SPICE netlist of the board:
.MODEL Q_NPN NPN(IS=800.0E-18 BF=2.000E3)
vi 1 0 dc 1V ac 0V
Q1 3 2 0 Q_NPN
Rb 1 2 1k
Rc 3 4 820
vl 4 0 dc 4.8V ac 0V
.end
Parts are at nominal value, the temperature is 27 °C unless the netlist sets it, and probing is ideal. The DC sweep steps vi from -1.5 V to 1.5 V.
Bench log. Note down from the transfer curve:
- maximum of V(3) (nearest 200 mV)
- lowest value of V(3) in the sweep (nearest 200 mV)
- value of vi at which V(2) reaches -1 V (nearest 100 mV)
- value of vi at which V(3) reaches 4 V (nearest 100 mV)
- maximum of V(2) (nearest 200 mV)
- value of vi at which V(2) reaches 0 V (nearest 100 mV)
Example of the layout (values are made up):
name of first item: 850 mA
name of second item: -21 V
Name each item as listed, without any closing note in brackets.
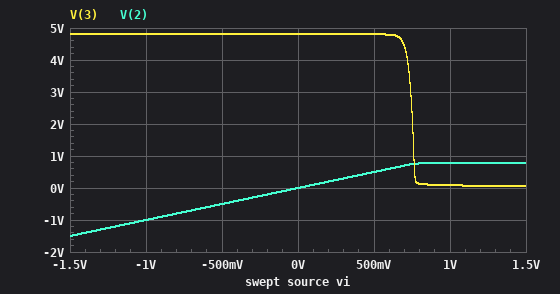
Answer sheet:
maximum of V(3): 4.8 V
lowest value of V(3) in the sweep: 0 V
value of vi at which V(2) reaches -1 V: -1.0 V
value of vi at which V(3) reaches 4 V: 700 mV
maximum of V(2): 800 mV
value of vi at which V(2) reaches 0 V: 0 V
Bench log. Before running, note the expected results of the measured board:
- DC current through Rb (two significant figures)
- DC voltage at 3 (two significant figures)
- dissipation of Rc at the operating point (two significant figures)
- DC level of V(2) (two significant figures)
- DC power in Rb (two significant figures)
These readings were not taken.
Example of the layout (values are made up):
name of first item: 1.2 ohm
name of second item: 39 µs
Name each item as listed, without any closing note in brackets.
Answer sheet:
DC current through Rb: 230 µA
DC voltage at 3: 85 mV
dissipation of Rc at the operating point: 27 mW
DC level of V(2): 770 mV
DC power in Rb: 54 µW
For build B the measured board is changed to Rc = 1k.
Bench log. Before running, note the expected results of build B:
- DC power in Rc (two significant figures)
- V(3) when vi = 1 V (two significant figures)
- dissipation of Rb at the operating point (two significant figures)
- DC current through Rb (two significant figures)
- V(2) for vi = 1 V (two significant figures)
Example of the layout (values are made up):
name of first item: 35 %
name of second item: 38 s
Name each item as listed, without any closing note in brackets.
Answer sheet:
DC power in Rc: 22 mW
V(3) when vi = 1 V: 80 mV
dissipation of Rb at the operating point: 56 µW
DC current through Rb: 240 µA
V(2) for vi = 1 V: 760 mV
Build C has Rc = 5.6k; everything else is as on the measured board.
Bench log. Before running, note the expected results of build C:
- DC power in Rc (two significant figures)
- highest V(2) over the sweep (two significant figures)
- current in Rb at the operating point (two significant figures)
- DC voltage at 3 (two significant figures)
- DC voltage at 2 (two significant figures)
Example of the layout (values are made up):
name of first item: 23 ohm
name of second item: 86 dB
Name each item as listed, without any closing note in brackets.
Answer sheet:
DC power in Rc: 4.0 mW
highest V(2) over the sweep: 740 mV
current in Rb at the operating point: 270 µA
DC voltage at 3: 42 mV
DC voltage at 2: 730 mV
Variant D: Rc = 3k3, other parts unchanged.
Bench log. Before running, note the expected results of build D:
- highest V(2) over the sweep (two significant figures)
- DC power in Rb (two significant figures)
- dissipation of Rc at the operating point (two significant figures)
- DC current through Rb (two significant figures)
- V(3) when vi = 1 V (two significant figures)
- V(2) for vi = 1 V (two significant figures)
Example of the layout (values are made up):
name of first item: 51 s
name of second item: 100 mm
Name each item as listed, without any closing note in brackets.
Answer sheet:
highest V(2) over the sweep: 750 mV
DC power in Rb: 69 µW
dissipation of Rc at the operating point: 6.8 mW
DC current through Rb: 260 µA
V(3) when vi = 1 V: 52 mV
V(2) for vi = 1 V: 740 mV
